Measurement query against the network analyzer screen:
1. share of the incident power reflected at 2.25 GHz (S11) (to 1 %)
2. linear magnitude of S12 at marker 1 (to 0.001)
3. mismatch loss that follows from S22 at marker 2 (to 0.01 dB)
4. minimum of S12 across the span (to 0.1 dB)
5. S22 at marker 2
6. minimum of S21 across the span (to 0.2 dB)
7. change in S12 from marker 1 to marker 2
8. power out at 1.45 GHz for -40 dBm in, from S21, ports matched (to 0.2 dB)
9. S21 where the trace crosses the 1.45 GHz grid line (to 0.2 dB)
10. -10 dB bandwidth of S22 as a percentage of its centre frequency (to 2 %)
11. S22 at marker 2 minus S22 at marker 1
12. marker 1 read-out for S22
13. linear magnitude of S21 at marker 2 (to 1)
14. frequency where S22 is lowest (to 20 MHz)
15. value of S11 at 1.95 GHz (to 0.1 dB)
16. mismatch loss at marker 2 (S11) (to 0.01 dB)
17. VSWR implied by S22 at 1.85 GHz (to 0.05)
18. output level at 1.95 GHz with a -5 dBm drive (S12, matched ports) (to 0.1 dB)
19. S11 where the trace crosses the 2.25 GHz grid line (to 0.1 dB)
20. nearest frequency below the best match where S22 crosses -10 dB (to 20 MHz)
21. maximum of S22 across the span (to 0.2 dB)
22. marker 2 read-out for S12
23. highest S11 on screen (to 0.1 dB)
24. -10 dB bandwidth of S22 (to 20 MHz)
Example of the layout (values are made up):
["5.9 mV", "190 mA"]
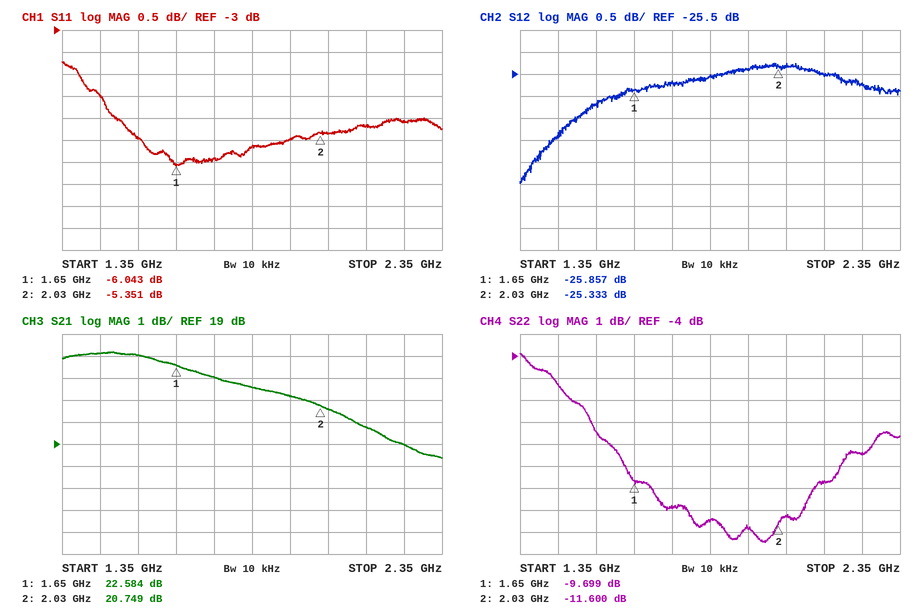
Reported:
["31 %", "0.051", "0.31 dB", "-28.0 dB", "-11.600 dB", "18.4 dB", "0.524 dB", "-16.8 dBm", "23.2 dB", "22 %", "-1.901 dB", "-9.699 dB", "11", "2.00 GHz", "-5.5 dB", "1.50 dB", "1.75", "-30.4 dBm", "-5.1 dB", "1.70 GHz", "-3.8 dB", "-25.333 dB", "-3.7 dB", "420 MHz"]
